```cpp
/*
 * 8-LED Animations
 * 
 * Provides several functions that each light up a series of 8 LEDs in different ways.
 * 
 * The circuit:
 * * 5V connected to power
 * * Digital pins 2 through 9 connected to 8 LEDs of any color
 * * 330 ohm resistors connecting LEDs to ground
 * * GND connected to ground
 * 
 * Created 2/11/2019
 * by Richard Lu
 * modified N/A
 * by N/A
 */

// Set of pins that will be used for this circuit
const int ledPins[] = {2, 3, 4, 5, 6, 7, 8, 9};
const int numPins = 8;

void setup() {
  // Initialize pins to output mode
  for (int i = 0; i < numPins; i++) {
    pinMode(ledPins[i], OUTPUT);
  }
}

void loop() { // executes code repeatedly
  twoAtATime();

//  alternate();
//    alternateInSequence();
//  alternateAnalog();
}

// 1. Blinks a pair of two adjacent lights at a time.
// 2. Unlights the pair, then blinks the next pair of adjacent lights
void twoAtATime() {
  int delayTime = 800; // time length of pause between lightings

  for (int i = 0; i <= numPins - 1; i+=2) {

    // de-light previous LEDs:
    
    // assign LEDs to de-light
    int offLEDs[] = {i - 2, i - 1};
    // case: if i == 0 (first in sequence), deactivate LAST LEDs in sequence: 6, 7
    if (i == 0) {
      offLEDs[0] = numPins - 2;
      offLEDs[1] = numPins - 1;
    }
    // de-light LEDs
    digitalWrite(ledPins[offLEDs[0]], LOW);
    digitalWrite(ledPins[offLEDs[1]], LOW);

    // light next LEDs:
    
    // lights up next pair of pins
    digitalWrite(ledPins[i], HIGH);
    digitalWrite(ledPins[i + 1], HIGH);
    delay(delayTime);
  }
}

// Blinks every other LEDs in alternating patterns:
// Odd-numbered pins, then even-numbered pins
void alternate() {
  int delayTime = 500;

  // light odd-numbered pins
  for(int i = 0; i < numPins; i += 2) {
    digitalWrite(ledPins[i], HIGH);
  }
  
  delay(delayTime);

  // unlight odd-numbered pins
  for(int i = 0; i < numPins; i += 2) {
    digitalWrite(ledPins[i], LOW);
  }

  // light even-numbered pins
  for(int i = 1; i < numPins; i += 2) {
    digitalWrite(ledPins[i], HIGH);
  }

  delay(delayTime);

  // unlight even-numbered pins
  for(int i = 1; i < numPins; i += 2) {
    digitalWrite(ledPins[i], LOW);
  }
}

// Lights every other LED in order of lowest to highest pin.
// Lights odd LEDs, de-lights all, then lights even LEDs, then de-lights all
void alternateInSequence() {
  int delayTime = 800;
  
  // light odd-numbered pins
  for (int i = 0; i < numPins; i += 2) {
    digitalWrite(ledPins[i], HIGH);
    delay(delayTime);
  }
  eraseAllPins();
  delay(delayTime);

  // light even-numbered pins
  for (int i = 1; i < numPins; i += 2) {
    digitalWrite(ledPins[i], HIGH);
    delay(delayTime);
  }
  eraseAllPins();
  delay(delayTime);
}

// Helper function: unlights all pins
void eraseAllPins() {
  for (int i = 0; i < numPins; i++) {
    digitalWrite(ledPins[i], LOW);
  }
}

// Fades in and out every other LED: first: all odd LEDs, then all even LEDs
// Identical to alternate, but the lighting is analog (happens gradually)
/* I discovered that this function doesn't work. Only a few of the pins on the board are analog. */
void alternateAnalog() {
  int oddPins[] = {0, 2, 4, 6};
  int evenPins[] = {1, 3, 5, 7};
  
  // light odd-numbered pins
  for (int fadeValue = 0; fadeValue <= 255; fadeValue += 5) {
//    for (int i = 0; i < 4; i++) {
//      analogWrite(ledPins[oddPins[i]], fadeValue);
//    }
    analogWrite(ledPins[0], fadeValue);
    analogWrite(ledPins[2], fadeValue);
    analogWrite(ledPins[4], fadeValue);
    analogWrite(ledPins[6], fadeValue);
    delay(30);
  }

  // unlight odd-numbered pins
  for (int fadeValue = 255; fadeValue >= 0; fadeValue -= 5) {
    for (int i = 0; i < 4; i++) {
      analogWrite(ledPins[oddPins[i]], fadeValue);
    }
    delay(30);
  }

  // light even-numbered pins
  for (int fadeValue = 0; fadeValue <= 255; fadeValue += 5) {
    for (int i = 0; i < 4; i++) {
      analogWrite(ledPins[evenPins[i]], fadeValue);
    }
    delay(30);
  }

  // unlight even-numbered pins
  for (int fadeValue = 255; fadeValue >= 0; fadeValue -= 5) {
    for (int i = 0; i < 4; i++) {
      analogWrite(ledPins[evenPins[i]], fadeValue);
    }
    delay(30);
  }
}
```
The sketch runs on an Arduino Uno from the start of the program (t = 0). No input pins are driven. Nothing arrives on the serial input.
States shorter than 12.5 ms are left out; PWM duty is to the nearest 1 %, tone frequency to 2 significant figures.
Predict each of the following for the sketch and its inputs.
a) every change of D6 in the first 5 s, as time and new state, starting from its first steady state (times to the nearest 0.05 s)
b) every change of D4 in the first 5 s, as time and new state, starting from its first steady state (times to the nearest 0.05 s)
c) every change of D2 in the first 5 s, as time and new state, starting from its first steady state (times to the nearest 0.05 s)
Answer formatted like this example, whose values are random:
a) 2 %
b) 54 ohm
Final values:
a) 0 s low; 1.6 s high; 2.4 s low; 4.8 s high
b) 0 s low; 0.8 s high; 1.6 s low; 4 s high; 4.8 s low
c) 0 s high; 0.8 s low; 3.2 s high; 4 s low
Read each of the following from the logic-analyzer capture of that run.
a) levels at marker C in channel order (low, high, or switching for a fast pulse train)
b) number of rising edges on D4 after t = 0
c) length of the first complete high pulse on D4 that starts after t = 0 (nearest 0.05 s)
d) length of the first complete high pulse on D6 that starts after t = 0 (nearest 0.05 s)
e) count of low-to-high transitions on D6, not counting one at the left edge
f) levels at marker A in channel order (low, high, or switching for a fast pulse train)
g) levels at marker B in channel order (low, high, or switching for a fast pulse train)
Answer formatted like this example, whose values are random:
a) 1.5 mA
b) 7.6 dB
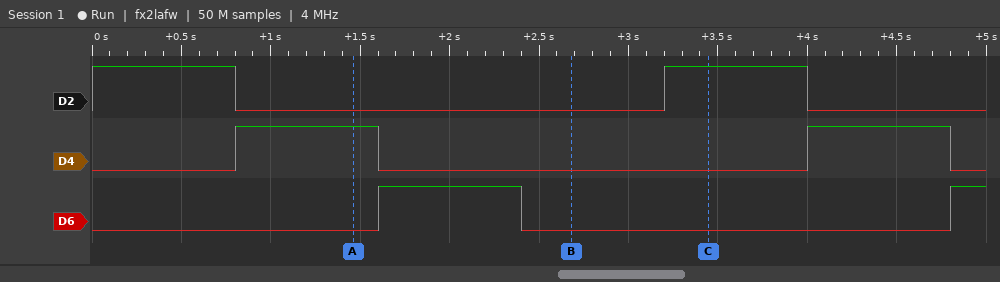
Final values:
a) D2 high, D4 low, D6 low
b) 2
c) 0.80 s
d) 0.80 s
e) 2
f) D2 low, D4 high, D6 low
g) D2 low, D4 low, D6 low
